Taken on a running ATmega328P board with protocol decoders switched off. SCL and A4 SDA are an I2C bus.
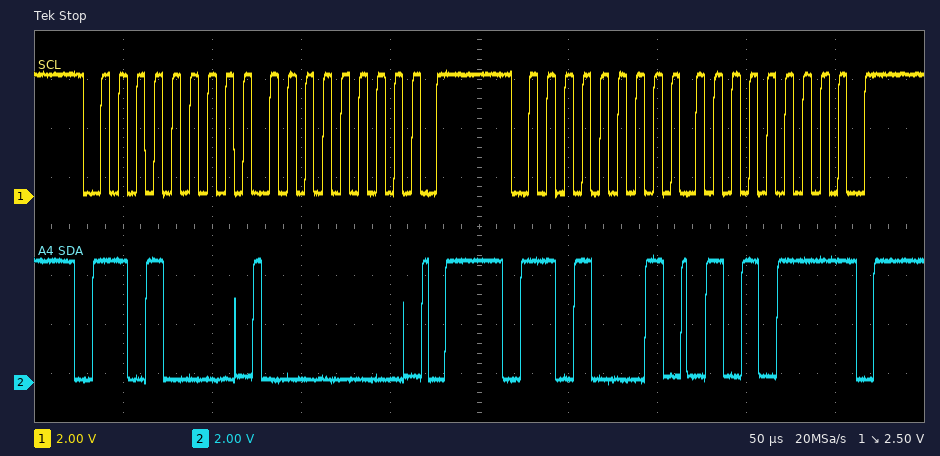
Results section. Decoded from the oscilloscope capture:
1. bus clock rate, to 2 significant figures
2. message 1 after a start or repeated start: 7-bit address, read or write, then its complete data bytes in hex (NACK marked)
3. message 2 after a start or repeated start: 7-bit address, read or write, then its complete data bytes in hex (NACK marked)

100 kHz
0x68 write: 00
0x68 read: 57 NACK
